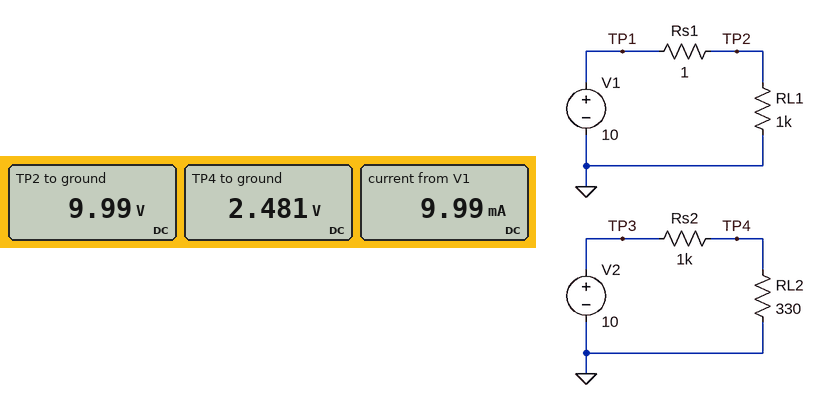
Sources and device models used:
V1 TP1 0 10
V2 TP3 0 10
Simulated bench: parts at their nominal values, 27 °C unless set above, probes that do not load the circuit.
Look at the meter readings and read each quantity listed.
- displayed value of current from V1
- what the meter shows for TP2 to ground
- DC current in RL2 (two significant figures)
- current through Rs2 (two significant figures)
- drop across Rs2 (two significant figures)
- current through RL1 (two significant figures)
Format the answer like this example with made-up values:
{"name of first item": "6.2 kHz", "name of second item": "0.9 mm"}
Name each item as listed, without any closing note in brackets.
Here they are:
{"displayed value of current from V1": "9.99 mA", "what the meter shows for TP2 to ground": "9.99 V", "DC current in RL2": "7.5 mA", "current through Rs2": "7.5 mA", "drop across Rs2": "7.5 V", "current through RL1": "10 mA"}
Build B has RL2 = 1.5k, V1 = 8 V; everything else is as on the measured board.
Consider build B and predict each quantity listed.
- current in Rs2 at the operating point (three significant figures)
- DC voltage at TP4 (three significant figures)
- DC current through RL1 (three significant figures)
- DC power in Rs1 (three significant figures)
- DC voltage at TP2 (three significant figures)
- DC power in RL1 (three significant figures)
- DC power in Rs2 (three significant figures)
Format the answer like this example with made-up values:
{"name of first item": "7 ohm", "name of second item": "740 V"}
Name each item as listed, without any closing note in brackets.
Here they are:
{"current in Rs2 at the operating point": "4.00 mA", "DC voltage at TP4": "6.00 V", "DC current through RL1": "7.99 mA", "DC power in Rs1": "63.9 µW", "DC voltage at TP2": "7.99 V", "DC power in RL1": "63.9 mW", "DC power in Rs2": "16.0 mW"}
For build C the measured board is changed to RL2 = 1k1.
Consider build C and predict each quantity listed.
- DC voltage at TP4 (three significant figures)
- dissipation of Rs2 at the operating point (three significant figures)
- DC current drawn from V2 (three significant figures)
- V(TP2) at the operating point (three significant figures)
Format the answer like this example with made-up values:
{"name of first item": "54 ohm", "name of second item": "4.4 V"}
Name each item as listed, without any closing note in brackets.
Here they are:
{"DC voltage at TP4": "5.24 V", "dissipation of Rs2 at the operating point": "22.7 mW", "DC current drawn from V2": "4.76 mA", "V(TP2) at the operating point": "9.99 V"}
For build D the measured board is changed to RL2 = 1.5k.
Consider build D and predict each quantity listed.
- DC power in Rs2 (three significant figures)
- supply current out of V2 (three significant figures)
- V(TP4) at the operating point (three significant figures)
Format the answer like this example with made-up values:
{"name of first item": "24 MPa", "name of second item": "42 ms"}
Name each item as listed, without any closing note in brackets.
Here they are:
{"DC power in Rs2": "16.0 mW", "supply current out of V2": "4.00 mA", "V(TP4) at the operating point": "6.00 V"}
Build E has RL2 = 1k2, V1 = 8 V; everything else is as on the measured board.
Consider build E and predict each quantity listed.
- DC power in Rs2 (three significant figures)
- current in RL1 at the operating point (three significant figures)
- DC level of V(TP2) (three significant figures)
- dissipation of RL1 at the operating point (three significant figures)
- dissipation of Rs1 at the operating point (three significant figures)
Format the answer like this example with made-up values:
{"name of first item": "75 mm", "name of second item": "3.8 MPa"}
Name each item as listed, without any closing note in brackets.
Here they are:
{"DC power in Rs2": "20.7 mW", "current in RL1 at the operating point": "7.99 mA", "DC level of V(TP2)": "7.99 V", "dissipation of RL1 at the operating point": "63.9 mW", "dissipation of Rs1 at the operating point": "63.9 µW"}
